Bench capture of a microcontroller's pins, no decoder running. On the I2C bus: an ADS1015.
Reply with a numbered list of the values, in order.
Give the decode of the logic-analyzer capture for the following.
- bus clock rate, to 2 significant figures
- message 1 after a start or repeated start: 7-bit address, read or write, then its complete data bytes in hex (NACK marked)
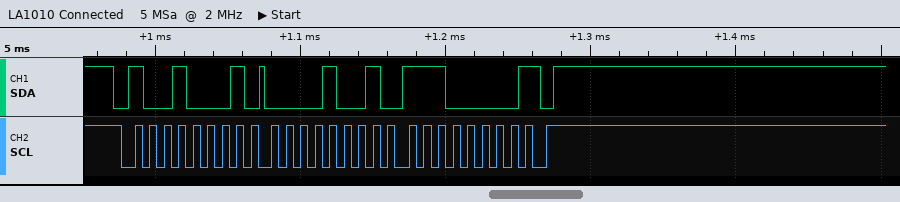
1. 100 kHz
2. 0x48 read: 09 E0 NACK
